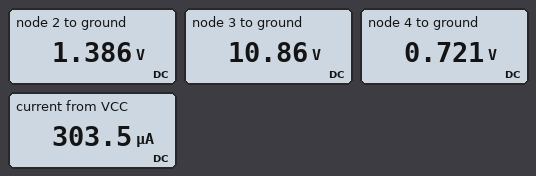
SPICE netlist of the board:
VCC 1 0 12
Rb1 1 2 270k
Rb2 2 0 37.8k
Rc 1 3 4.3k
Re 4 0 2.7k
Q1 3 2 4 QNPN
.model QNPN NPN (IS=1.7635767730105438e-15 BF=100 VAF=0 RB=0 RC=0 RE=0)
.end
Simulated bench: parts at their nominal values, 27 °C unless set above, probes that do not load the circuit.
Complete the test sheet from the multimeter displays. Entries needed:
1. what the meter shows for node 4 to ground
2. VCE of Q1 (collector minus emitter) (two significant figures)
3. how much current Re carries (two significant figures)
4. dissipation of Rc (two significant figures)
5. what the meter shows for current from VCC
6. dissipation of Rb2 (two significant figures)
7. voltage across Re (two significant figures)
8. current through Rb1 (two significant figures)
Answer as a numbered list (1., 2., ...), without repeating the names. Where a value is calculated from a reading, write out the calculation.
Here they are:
1. 0.721 V
2. 10.86 V - 721 mV = 10 V
3. (721 mV) / 2.7 kΩ = 270 µA
4. (12 V - 10.86 V)^2 / 4.3 kΩ = 300 µW
5. 303.5 µA
6. (1.386 V)^2 / 37.8 kΩ = 51 µW
7. 721 mV = 720 mV
8. (12 V - 1.386 V) / 270 kΩ = 39 µA
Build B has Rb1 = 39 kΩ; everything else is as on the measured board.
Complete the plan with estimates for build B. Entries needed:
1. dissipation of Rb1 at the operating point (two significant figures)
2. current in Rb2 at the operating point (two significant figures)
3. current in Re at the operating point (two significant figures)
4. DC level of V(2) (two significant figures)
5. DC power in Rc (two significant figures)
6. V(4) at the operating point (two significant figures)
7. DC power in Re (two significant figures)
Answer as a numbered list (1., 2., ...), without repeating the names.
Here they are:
1. 1.1 mW
2. 140 µA
3. 1.7 mA
4. 5.3 V
5. 12 mW
6. 4.6 V
7. 7.9 mW
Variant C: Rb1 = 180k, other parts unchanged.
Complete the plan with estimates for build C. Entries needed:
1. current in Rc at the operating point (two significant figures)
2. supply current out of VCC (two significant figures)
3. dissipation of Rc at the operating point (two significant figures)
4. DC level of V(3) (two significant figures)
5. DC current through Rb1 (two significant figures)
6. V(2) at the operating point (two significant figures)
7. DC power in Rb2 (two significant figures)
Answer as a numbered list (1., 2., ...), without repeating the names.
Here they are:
1. 460 µA
2. 520 µA
3. 920 µW
4. 10 V
5. 56 µA
6. 1.9 V
7. 99 µW
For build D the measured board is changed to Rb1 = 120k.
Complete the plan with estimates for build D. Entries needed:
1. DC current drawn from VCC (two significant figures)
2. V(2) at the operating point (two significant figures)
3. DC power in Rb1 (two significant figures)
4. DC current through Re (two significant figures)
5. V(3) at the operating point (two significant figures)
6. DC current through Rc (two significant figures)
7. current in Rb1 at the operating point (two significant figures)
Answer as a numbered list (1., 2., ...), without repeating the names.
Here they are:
1. 800 µA
2. 2.7 V
3. 730 µW
4. 730 µA
5. 8.9 V
6. 720 µA
7. 78 µA
